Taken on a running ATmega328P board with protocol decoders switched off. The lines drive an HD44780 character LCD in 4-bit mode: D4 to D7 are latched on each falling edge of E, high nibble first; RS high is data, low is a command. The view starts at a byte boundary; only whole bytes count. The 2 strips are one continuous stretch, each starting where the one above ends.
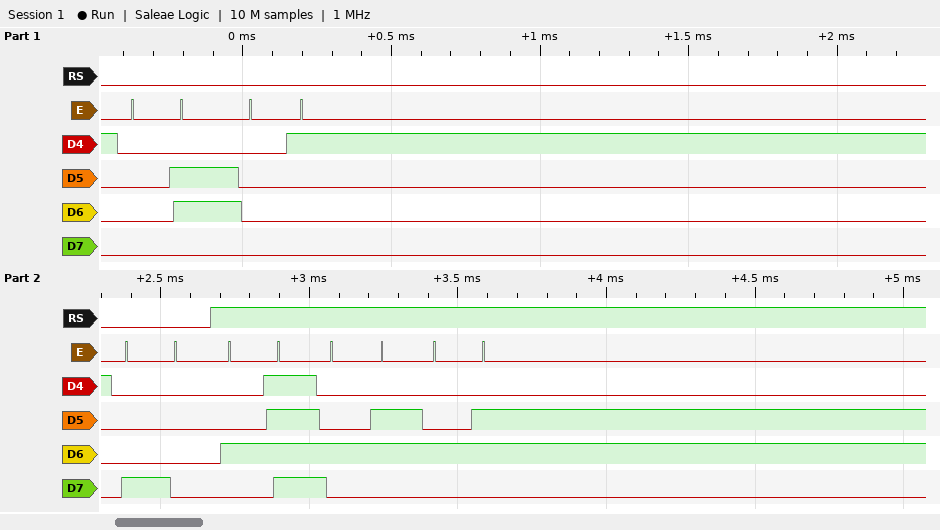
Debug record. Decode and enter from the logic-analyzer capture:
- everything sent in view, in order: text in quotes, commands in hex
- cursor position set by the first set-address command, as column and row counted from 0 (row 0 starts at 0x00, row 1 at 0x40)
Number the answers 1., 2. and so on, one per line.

1. 0x06 0x01 0x80 "OFF"
2. column 0, row 0
